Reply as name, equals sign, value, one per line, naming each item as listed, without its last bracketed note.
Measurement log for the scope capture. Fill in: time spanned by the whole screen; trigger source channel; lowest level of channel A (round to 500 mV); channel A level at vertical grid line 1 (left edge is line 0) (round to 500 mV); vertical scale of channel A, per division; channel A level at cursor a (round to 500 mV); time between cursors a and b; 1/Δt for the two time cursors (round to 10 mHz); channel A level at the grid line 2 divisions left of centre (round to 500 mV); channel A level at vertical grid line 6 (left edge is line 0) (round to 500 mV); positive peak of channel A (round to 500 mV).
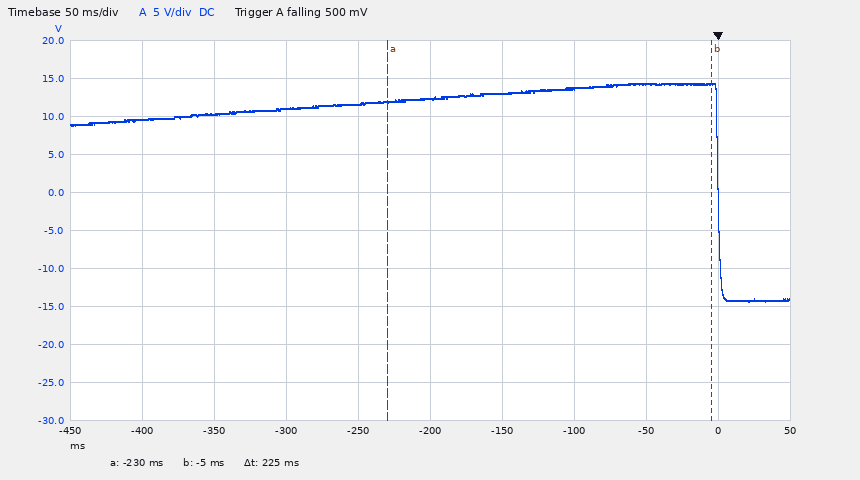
time spanned by the whole screen = 500 ms
trigger source channel = channel A
lowest level of channel A = -14.5 V
channel A level at vertical grid line 1 (left edge is line 0) = 9.5 V
vertical scale of channel A, per division = 5 V
channel A level at cursor a = 12.0 V
time between cursors a and b = 225 ms
1/Δt for the two time cursors = 4.44 Hz
channel A level at the grid line 2 divisions left of centre = 11.0 V
channel A level at vertical grid line 6 (left edge is line 0) = 13.0 V
positive peak of channel A = 14.5 V
